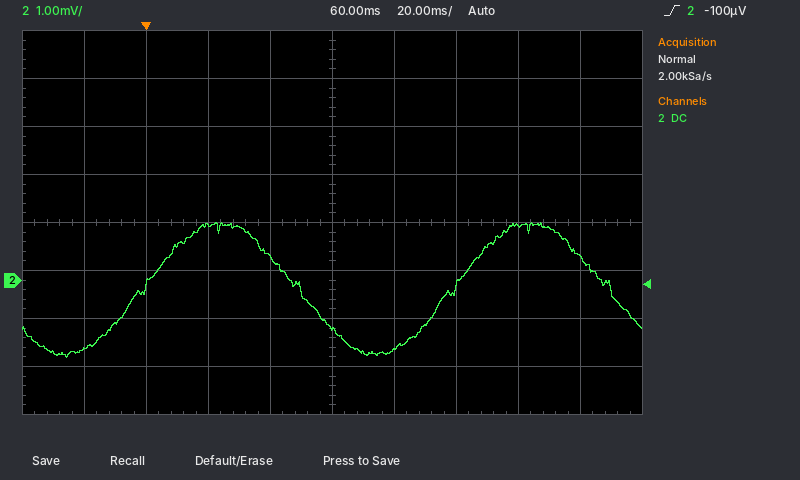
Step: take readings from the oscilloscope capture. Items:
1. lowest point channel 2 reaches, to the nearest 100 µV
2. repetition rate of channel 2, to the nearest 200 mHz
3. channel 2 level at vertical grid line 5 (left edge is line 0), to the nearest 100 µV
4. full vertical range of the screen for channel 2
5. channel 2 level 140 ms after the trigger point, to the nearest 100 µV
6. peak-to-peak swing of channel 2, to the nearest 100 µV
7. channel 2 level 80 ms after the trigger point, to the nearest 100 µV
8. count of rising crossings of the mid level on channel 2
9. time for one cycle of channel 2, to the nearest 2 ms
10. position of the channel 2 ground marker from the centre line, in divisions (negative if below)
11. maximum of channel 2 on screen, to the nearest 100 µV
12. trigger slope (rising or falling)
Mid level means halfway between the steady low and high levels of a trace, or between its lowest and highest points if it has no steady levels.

-1.6 mV
10.0 Hz
-1.0 mV
8 mV
500 µV
2.8 mV
-1.4 mV
2
100 ms
-1.2 div
1.2 mV
rising
